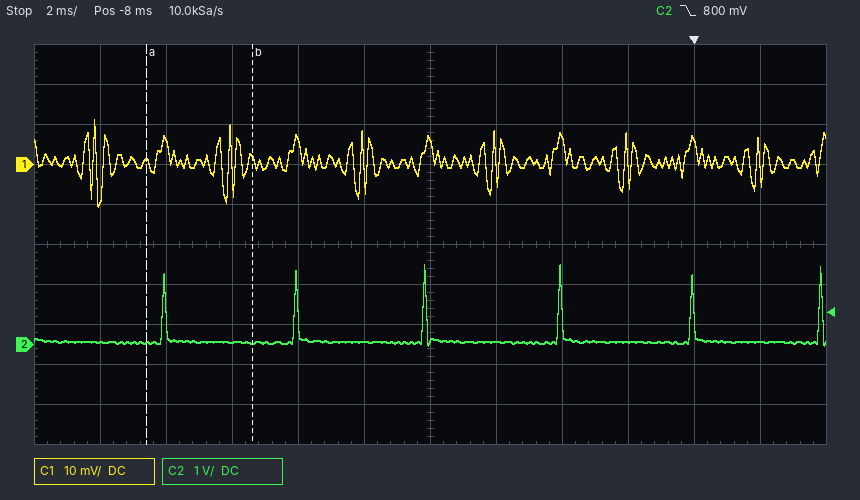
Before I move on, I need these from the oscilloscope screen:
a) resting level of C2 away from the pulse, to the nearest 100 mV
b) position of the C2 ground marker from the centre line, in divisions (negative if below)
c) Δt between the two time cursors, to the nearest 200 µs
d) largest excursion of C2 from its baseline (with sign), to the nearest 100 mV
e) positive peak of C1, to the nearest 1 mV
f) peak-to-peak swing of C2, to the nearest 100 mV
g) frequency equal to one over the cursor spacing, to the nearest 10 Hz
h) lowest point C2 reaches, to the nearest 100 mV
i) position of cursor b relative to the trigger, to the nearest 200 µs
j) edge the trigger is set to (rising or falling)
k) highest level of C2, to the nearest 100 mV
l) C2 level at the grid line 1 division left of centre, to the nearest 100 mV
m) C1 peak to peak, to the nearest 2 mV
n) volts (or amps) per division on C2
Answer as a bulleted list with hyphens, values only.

- 100 mV
- -2.5 div
- 3.2 ms
- +1.9 V
- 11 mV
- 2.0 V
- 310 Hz
- 0.0 V
- -13.4 ms
- falling
- 2.0 V
- 100 mV
- 22 mV
- 1 V
